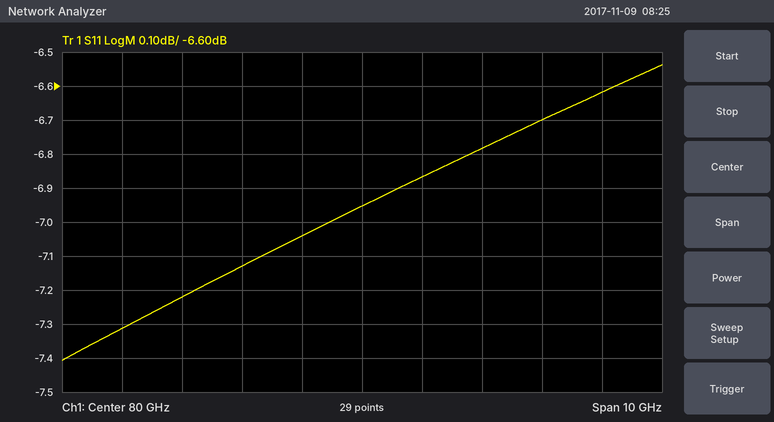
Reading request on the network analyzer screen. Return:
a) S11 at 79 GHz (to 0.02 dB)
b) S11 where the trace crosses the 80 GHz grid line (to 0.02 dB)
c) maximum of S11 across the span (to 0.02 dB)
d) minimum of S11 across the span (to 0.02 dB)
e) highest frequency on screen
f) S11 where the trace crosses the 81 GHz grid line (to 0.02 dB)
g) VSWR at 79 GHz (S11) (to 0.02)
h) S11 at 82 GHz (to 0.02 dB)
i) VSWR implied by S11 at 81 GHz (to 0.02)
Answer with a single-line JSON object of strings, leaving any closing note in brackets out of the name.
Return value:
{"S11 at 79 GHz": "-7.04 dB", "S11 where the trace crosses the 80 GHz grid line": "-6.96 dB", "maximum of S11 across the span": "-6.54 dB", "minimum of S11 across the span": "-7.40 dB", "highest frequency on screen": "85 GHz", "S11 where the trace crosses the 81 GHz grid line": "-6.86 dB", "VSWR at 79 GHz (S11)": "2.60", "S11 at 82 GHz": "-6.78 dB", "VSWR implied by S11 at 81 GHz": "2.66"}
